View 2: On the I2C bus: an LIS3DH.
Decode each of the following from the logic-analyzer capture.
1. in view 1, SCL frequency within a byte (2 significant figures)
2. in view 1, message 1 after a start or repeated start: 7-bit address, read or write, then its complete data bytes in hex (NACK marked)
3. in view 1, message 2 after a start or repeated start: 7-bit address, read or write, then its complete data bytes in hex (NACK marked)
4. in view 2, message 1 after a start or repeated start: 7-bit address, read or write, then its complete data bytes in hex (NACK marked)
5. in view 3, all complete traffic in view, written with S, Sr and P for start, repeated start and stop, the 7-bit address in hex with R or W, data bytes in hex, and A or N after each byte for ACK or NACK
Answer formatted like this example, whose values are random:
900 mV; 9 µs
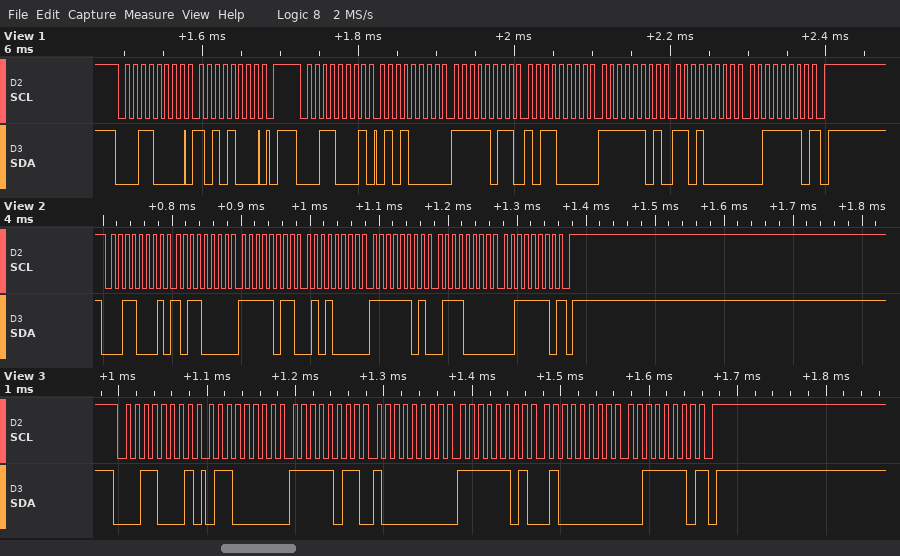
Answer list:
100 kHz; 0x18 write: A8; 0x18 read: 50 FB B0 FD D0 3E NACK; 0x18 read: B0 FB 50 FD 70 3E NACK; S 18R A 60 A FB A 80 A FD A 40 A 3E N P
